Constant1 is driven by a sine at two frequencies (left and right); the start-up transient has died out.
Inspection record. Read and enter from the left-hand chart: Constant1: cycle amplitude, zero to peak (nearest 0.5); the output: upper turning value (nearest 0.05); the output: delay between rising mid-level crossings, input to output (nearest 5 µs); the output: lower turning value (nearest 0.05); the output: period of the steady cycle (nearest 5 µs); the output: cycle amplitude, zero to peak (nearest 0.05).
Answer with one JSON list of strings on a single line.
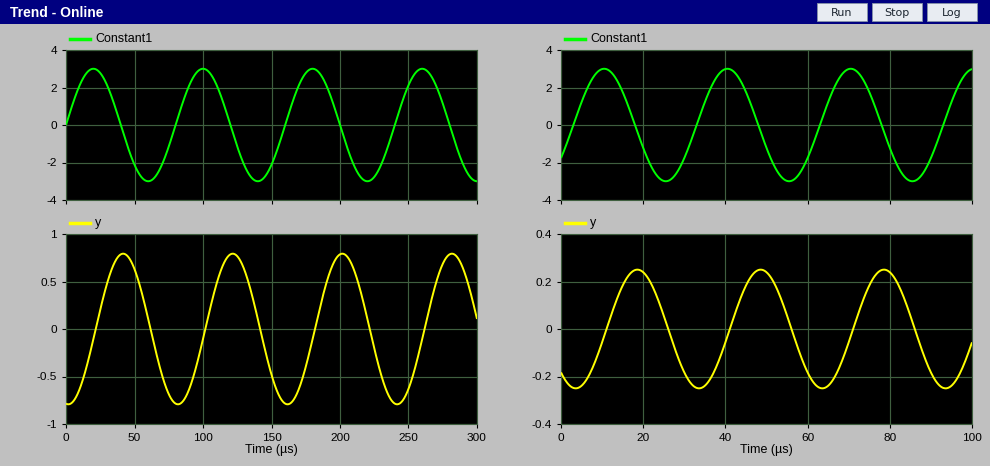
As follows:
["3.0", "0.80", "20 µs", "-0.80", "80 µs", "0.80"]
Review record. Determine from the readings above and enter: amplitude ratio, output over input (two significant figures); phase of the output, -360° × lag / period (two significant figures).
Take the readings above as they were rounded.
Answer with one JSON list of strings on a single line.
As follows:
["0.27", "-90°"]
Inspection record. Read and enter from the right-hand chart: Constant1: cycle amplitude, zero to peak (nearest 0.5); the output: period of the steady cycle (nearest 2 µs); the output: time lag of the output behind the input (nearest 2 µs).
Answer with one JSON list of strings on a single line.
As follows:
["3.0", "30 µs", "8 µs"]
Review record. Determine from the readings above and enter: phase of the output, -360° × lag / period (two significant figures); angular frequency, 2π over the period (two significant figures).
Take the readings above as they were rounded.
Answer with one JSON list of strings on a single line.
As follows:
["-96°", "0.21 rad/µs"]
